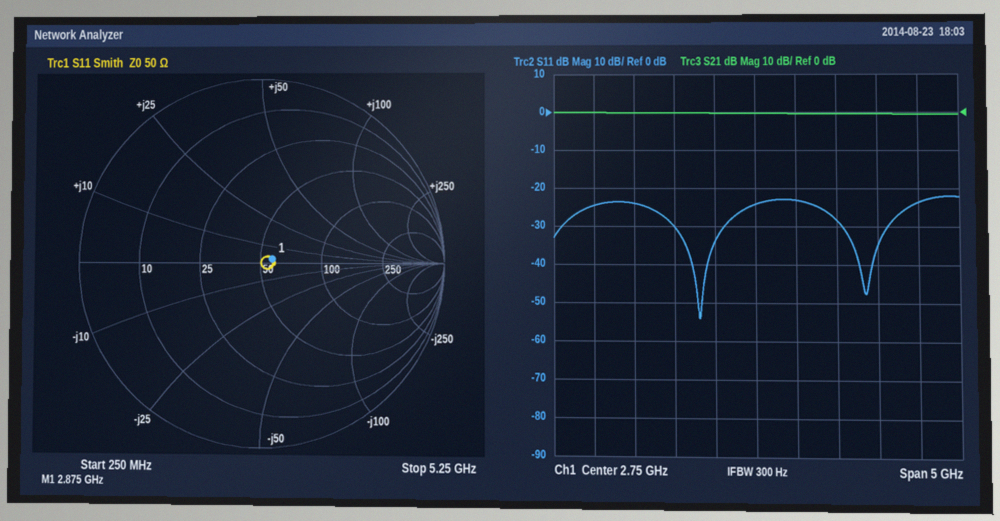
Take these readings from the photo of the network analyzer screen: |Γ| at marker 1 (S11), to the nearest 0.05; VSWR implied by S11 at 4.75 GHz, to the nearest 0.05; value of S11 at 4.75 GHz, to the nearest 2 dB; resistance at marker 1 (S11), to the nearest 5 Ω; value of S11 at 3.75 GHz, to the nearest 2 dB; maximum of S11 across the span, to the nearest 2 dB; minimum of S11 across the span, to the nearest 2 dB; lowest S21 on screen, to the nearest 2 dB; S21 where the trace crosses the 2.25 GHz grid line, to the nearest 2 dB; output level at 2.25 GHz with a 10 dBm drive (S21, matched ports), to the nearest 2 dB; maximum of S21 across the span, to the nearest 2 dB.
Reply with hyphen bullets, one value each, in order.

- 0.05
- 1.15
- -24 dB
- 55 Ω
- -28 dB
- -22 dB
- -54 dB
- 0 dB
- 0 dB
- 10 dBm
- 0 dB
